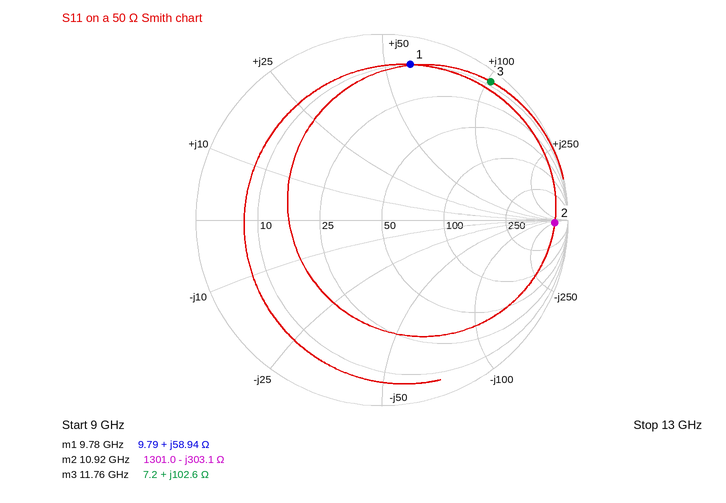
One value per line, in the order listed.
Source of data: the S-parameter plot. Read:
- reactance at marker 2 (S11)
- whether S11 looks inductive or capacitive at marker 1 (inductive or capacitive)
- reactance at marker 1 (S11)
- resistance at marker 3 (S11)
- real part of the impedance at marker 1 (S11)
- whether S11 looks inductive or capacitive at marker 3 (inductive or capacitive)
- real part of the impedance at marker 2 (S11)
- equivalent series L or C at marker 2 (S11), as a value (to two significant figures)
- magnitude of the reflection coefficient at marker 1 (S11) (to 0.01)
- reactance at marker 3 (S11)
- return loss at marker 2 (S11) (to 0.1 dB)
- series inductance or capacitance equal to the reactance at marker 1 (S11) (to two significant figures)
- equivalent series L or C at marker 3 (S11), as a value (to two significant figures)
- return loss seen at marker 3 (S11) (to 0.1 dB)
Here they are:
-303.1 Ω
inductive
+58.94 Ω
7.2 Ω
9.79 Ω
inductive
1301.0 Ω
48 fF
0.85
+102.6 Ω
0.6 dB
960 pH
1.4 nH
0.5 dB
